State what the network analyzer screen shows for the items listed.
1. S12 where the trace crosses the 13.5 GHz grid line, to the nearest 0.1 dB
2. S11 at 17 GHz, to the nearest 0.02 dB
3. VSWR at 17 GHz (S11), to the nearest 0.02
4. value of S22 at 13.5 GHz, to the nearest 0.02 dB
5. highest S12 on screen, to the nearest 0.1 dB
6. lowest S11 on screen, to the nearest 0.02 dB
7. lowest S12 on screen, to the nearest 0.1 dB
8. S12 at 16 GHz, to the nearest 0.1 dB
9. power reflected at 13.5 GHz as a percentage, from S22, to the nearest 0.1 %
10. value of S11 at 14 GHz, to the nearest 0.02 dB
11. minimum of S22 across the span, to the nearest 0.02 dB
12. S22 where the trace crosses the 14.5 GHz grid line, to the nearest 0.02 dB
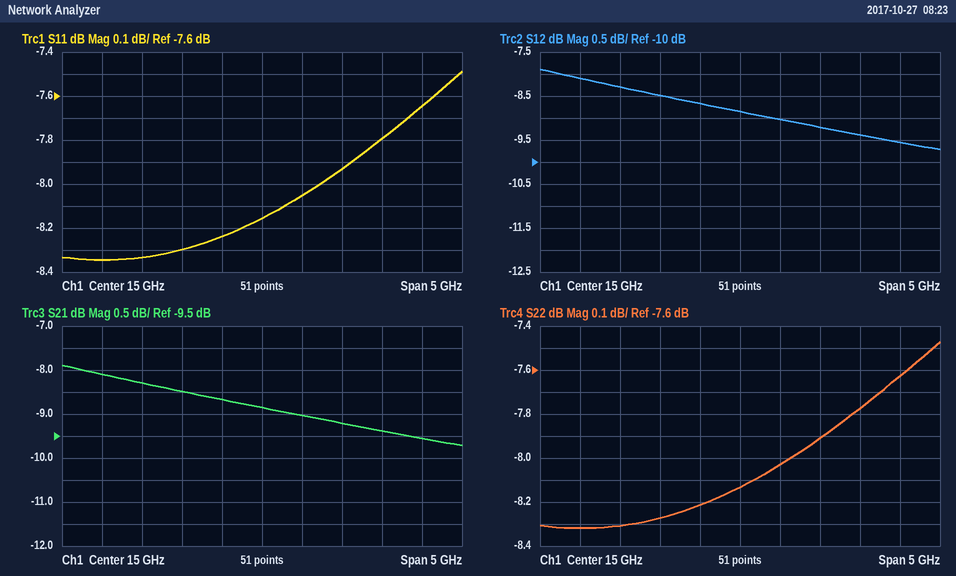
-8.3 dB
-7.64 dB
2.42
-8.30 dB
-7.9 dB
-8.34 dB
-9.7 dB
-9.2 dB
14.8 %
-8.30 dB
-8.32 dB
-8.22 dB
